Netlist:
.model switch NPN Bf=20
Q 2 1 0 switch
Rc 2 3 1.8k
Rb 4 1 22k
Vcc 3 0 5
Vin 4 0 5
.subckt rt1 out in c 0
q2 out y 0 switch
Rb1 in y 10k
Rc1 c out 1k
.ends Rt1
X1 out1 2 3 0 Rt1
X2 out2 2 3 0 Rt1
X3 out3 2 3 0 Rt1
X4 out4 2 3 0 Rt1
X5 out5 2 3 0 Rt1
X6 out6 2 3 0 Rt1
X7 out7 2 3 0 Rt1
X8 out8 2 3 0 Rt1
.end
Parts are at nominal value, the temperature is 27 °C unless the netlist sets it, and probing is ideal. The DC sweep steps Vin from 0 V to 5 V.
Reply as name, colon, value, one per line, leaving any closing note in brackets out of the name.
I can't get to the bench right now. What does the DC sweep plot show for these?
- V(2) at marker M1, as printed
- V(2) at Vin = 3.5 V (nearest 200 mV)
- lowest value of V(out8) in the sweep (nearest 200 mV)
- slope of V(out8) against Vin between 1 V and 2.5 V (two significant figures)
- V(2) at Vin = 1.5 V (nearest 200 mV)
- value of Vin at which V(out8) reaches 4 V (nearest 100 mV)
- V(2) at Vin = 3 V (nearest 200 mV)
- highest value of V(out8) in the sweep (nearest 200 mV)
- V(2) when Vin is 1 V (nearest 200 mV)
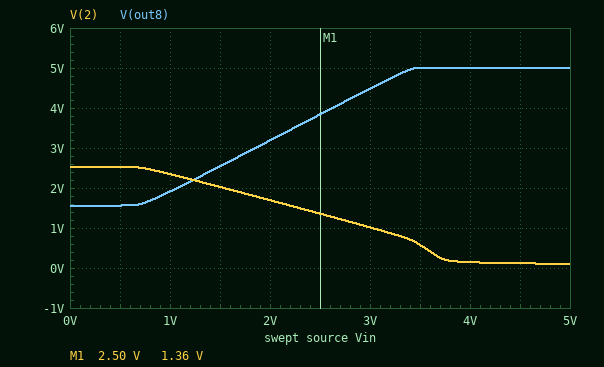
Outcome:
V(2) at marker M1, as printed: 1.36 V
V(2) at Vin = 3.5 V: 600 mV
lowest value of V(out8) in the sweep: 1.6 V
slope of V(out8) against Vin between 1 V and 2.5 V: 1.3 V/V
V(2) at Vin = 1.5 V: 2.0 V
value of Vin at which V(out8) reaches 4 V: 2.6 V
V(2) at Vin = 3 V: 1.0 V
highest value of V(out8) in the sweep: 5.0 V
V(2) when Vin is 1 V: 2.4 V
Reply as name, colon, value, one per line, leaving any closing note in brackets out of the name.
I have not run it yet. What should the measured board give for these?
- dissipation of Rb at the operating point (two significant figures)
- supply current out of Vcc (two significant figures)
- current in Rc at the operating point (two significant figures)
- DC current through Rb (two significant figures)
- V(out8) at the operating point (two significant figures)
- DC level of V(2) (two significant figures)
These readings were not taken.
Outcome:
dissipation of Rb at the operating point: 800 µW
supply current out of Vcc: 2.7 mA
current in Rc at the operating point: 2.7 mA
DC current through Rb: 190 µA
V(out8) at the operating point: 5.0 V
DC level of V(2): 100 mV
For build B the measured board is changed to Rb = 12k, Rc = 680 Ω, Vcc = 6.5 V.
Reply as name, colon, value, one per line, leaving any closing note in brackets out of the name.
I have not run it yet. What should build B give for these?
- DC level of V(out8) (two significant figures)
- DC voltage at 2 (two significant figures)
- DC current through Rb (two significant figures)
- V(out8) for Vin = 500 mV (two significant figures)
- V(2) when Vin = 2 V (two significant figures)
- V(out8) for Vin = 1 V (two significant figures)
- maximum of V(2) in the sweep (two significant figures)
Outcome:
DC level of V(out8): 5.2 V
DC voltage at 2: 1.4 V
DC current through Rb: 350 µA
V(out8) for Vin = 500 mV: 130 mV
V(2) when Vin = 2 V: 3.6 V
V(out8) for Vin = 1 V: 140 mV
maximum of V(2) in the sweep: 4.5 V
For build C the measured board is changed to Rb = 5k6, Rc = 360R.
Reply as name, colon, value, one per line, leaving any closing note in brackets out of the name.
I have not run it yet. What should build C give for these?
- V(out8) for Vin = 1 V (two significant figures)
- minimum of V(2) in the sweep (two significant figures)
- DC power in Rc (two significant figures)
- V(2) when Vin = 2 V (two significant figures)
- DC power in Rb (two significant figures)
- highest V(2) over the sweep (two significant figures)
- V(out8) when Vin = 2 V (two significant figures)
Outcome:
V(out8) for Vin = 1 V: 120 mV
minimum of V(2) in the sweep: 140 mV
DC power in Rc: 66 mW
V(2) when Vin = 2 V: 2.9 V
DC power in Rb: 3.1 mW
highest V(2) over the sweep: 4.1 V
V(out8) when Vin = 2 V: 870 mV
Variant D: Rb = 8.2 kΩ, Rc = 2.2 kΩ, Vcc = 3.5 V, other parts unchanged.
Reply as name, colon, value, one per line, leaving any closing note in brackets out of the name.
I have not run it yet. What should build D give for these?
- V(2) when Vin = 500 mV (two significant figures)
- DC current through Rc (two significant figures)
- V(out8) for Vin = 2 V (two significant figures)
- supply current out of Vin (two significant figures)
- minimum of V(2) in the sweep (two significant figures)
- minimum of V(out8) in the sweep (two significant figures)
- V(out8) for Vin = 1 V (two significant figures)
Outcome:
V(2) when Vin = 500 mV: 1.8 V
DC current through Rc: 1.6 mA
V(out8) for Vin = 2 V: 3.5 V
supply current out of Vin: 510 µA
minimum of V(2) in the sweep: 46 mV
minimum of V(out8) in the sweep: 1.5 V
V(out8) for Vin = 1 V: 2.5 V
